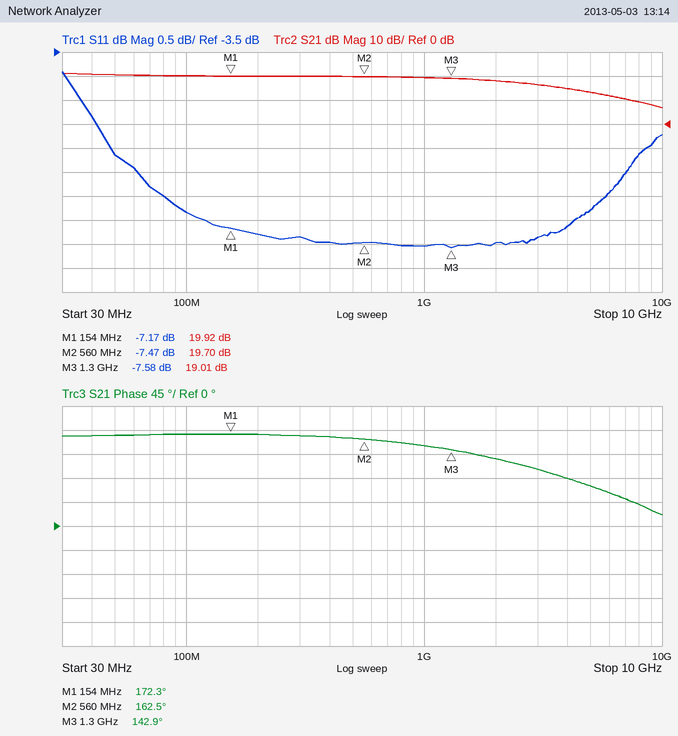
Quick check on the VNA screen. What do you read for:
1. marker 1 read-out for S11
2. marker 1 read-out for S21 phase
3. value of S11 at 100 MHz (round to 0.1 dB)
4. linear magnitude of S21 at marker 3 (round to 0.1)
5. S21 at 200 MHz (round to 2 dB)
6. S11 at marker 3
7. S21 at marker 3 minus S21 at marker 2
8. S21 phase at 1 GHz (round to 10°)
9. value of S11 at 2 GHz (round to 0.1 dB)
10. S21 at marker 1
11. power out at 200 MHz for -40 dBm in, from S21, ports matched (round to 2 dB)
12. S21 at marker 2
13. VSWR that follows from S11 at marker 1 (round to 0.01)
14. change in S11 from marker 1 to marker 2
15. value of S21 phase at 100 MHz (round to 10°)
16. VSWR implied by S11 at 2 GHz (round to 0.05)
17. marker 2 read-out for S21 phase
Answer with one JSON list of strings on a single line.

["-7.17 dB", "172.3°", "-6.8 dB", "8.9", "20 dB", "-7.58 dB", "-0.69 dB", "150°", "-7.5 dB", "19.92 dB", "-20 dBm", "19.70 dB", "2.56", "-0.30 dB", "170°", "2.45", "162.5°"]
